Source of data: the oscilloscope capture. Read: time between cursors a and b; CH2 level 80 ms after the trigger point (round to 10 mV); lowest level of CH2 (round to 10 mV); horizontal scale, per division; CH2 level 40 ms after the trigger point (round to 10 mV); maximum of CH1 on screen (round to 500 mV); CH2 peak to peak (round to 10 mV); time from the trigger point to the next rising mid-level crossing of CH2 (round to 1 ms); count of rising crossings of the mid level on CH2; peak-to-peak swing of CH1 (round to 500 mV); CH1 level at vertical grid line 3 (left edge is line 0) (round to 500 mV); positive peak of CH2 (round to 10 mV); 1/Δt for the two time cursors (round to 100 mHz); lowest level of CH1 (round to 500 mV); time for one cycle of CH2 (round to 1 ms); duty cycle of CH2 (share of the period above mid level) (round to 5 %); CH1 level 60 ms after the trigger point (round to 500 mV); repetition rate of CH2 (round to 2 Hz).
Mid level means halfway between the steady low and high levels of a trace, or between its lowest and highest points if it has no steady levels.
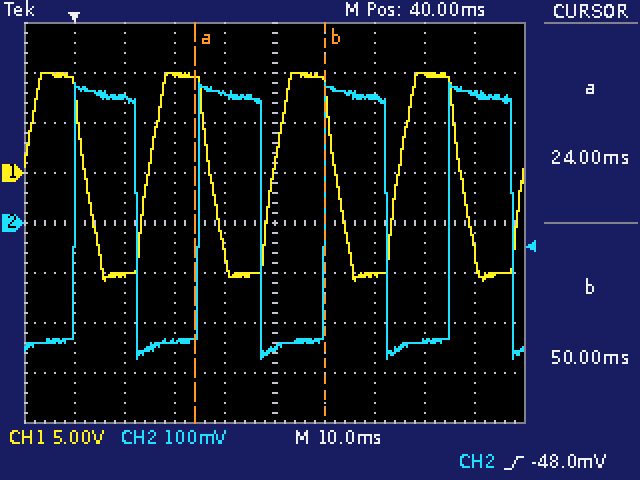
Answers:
26 ms
260 mV
-270 mV
10 ms
-250 mV
10.0 V
550 mV
25 ms
4
21.0 V
10.0 V
280 mV
38.5 Hz
-11.0 V
25 ms
50 %
-10.0 V
40 Hz
